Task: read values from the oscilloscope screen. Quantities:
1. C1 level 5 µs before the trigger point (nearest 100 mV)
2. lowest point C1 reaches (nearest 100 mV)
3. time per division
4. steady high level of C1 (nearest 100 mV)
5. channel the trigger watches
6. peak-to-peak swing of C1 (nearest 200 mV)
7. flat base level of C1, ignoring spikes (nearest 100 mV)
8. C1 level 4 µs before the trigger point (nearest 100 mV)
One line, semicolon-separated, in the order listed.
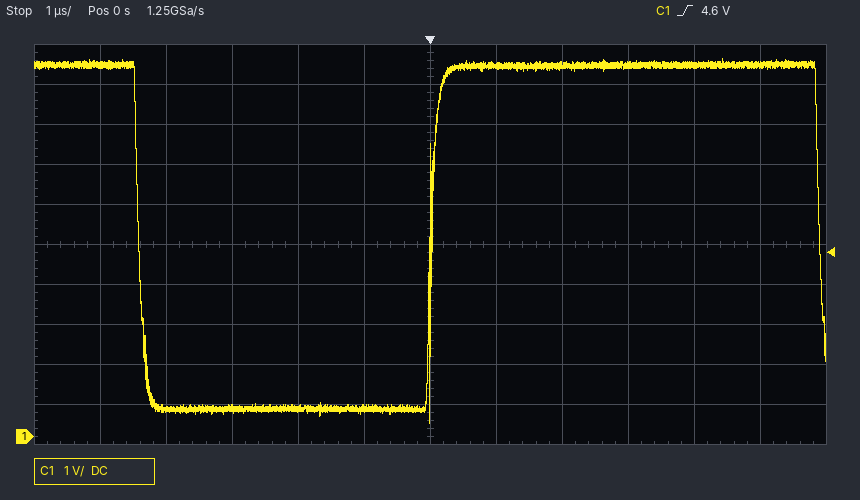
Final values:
9.3 V; 300 mV; 1 µs; 9.3 V; C1; 9.2 V; 700 mV; 700 mV
